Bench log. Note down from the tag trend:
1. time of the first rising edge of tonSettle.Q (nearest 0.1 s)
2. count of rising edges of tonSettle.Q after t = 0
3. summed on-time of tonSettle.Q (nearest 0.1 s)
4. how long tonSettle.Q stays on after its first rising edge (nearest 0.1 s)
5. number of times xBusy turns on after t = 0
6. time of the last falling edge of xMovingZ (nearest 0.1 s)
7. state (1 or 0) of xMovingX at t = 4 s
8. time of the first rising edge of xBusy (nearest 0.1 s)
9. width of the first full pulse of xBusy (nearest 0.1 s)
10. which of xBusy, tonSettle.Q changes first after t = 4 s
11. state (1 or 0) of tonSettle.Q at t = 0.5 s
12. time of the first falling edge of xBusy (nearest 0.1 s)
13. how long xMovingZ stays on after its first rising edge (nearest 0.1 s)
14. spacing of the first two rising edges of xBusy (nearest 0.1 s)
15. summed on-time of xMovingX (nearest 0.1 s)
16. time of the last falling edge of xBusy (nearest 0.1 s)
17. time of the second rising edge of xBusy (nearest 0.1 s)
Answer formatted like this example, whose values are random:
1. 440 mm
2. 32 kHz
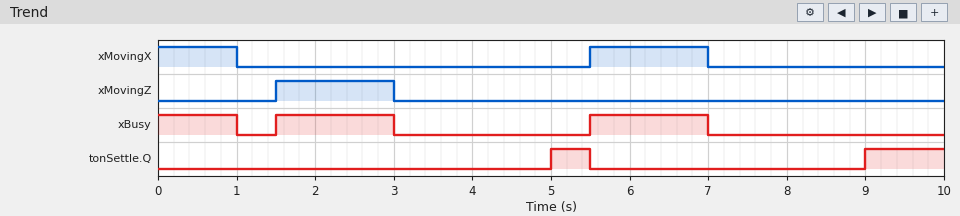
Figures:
1. 5.0 s
2. 2
3. 1.5 s
4. 0.5 s
5. 2
6. 3.0 s
7. 0
8. 1.5 s
9. 1.5 s
10. tonSettle.Q
11. 0
12. 1.0 s
13. 1.5 s
14. 4.0 s
15. 2.5 s
16. 7.0 s
17. 5.5 s
